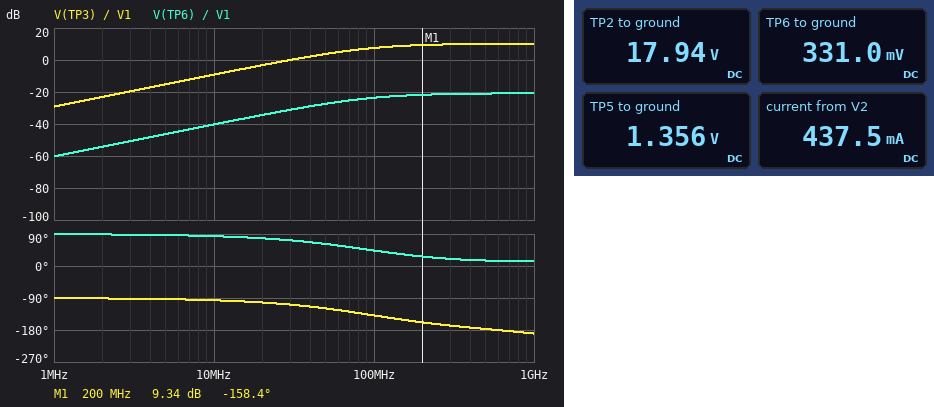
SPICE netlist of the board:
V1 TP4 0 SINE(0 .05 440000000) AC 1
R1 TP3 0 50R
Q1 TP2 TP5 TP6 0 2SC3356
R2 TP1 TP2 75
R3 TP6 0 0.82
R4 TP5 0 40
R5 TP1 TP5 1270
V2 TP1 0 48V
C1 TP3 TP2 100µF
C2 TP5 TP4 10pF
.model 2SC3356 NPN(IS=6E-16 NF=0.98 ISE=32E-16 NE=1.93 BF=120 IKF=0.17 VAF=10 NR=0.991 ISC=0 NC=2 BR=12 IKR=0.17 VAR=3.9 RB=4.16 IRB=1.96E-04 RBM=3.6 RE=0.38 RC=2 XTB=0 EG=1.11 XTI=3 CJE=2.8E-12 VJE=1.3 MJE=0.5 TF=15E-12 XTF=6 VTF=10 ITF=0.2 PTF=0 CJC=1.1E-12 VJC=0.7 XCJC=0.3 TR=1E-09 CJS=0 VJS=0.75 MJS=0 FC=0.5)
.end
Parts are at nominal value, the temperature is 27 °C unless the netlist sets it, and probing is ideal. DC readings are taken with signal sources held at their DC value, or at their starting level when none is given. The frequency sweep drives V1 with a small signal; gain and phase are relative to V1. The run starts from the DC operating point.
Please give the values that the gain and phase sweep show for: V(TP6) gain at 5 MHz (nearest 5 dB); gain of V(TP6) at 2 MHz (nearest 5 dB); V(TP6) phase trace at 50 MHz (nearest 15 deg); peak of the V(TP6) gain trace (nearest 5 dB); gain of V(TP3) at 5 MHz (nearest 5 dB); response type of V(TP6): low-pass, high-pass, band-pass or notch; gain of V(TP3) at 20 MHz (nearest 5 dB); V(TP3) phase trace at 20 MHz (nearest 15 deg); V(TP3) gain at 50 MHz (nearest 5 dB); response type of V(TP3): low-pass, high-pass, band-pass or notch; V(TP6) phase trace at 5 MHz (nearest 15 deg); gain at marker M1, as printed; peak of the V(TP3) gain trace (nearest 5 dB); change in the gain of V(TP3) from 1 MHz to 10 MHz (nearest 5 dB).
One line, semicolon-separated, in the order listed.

-45 dB; -55 dB; 60 deg; -20 dB; -15 dB; high-pass; -5 dB; -105 deg; 5 dB; high-pass; 90 deg; 9.34 dB; 10 dB; 20 dB
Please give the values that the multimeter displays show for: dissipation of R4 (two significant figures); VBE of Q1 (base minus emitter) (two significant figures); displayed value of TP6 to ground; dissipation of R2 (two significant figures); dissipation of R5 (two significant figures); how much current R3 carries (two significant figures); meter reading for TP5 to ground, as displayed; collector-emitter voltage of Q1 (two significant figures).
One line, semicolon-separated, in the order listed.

46 mW; 1.0 V; 331.0 mV; 12 W; 1.7 W; 400 mA; 1.356 V; 18 V
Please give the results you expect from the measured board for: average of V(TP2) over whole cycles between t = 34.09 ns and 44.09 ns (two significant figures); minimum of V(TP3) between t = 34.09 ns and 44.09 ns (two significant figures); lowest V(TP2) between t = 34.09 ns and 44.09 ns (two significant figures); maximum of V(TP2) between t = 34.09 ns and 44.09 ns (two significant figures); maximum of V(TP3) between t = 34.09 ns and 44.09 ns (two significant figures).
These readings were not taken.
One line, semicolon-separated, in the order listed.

18 V; -160 mV; 18 V; 18 V; 160 mV
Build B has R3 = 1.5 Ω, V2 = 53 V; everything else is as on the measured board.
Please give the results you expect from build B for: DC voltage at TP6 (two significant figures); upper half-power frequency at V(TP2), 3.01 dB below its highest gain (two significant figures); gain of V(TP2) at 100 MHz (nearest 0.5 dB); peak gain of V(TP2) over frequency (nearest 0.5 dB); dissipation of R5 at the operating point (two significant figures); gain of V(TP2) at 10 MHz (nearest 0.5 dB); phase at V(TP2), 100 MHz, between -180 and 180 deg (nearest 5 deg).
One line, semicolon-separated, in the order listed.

560 mV; 5.9 GHz; 8.0 dB; 12.5 dB; 2.1 W; -10.5 dB; -125 deg
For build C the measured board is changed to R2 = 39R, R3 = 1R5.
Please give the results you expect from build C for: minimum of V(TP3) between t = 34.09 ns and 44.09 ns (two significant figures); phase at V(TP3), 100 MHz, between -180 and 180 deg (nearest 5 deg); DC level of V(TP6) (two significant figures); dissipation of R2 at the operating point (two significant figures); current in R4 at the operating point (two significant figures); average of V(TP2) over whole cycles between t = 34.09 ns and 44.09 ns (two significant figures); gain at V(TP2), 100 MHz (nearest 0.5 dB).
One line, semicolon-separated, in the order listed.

-200 mV; -120 deg; 470 mV; 3.9 W; 36 mA; 36 V; 6.5 dB
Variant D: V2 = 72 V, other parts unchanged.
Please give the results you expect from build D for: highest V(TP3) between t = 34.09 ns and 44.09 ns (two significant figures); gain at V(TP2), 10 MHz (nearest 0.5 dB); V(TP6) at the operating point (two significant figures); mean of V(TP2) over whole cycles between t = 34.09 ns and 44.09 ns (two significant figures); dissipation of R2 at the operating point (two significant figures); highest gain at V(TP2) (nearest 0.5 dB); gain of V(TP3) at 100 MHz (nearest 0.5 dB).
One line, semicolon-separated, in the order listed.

92 mV; -13.5 dB; 620 mV; 16 V; 42 W; 5.5 dB; 3.0 dB
